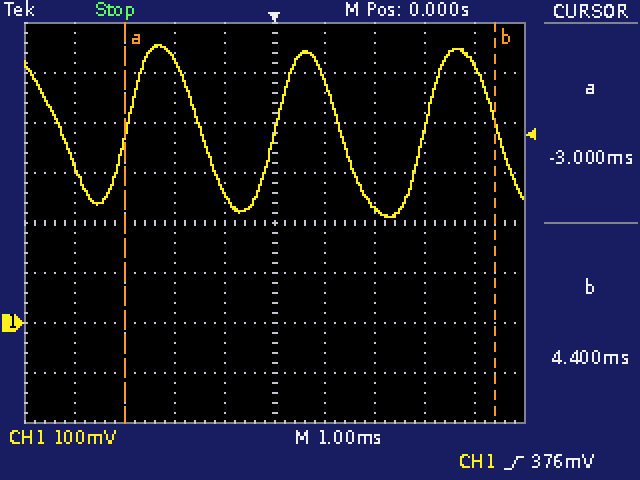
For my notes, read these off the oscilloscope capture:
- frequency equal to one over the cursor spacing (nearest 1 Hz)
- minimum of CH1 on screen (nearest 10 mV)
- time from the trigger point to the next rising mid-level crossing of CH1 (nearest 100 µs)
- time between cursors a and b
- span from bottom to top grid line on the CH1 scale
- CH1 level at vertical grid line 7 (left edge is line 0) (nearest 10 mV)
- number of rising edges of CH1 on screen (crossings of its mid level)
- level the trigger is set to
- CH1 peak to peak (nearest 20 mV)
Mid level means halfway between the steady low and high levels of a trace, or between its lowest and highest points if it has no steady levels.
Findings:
135 Hz
210 mV
3.0 ms
7.4 ms
800 mV
230 mV
3
376 mV
340 mV
